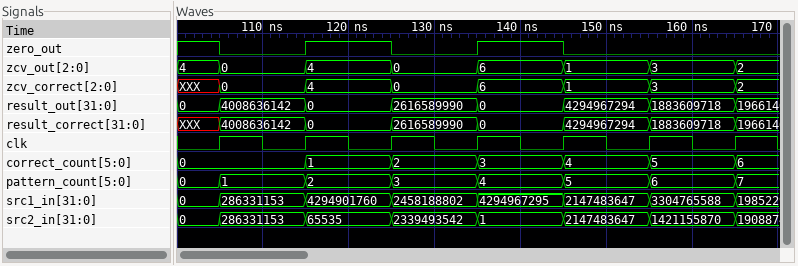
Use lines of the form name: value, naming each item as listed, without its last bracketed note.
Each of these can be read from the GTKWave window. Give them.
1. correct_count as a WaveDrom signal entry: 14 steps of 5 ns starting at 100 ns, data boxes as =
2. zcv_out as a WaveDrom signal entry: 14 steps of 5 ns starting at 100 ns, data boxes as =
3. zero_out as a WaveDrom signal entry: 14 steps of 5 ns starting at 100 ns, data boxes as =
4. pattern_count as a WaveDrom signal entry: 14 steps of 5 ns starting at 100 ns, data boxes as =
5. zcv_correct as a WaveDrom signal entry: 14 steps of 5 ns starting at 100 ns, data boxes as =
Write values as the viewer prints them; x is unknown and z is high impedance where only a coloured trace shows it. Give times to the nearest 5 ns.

correct_count as a WaveDrom signal entry: 14 steps of 5 ns starting at 100 ns, data boxes as =: {name: 'correct_count', wave: '=..=.=.=.=.=.=', data: '0 1 2 3 4 5 6'}
zcv_out as a WaveDrom signal entry: 14 steps of 5 ns starting at 100 ns, data boxes as =: {name: 'zcv_out', wave: '==.=.=.=.=.=.=', data: '4 0 4 0 6 1 3 2'}
zero_out as a WaveDrom signal entry: 14 steps of 5 ns starting at 100 ns, data boxes as =: {name: 'zero_out', wave: '10.1.0.1.0....'}
pattern_count as a WaveDrom signal entry: 14 steps of 5 ns starting at 100 ns, data boxes as =: {name: 'pattern_count', wave: '==.=.=.=.=.=.=', data: '0 1 2 3 4 5 6 7'}
zcv_correct as a WaveDrom signal entry: 14 steps of 5 ns starting at 100 ns, data boxes as =: {name: 'zcv_correct', wave: 'x=.=.=.=.=.=.=', data: '0 4 0 6 1 3 2'}
